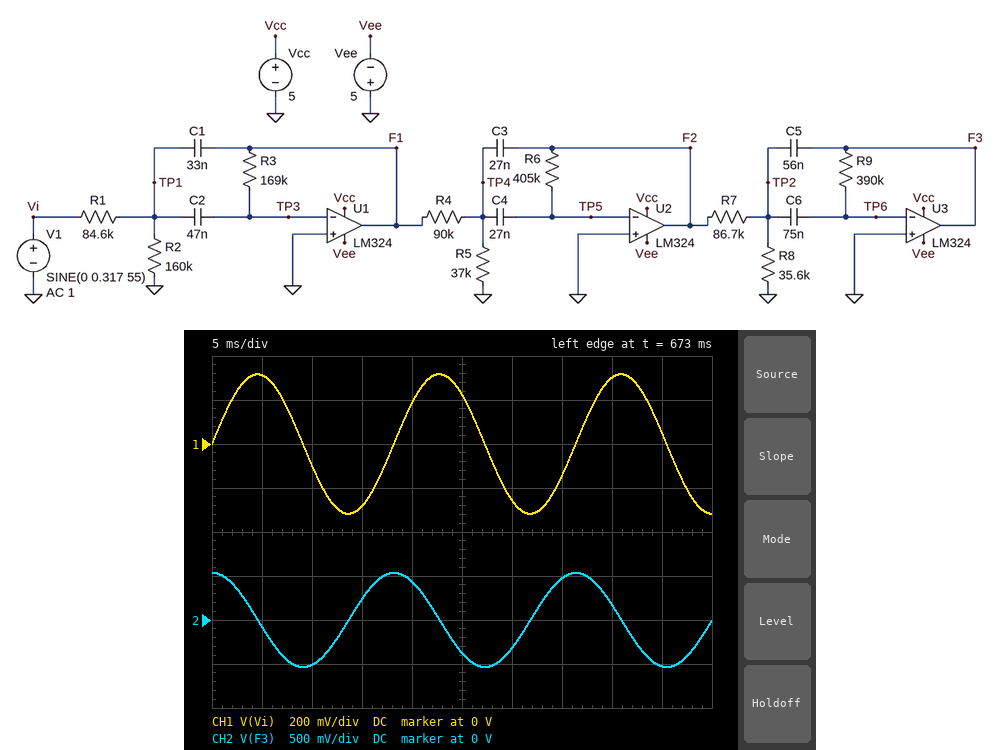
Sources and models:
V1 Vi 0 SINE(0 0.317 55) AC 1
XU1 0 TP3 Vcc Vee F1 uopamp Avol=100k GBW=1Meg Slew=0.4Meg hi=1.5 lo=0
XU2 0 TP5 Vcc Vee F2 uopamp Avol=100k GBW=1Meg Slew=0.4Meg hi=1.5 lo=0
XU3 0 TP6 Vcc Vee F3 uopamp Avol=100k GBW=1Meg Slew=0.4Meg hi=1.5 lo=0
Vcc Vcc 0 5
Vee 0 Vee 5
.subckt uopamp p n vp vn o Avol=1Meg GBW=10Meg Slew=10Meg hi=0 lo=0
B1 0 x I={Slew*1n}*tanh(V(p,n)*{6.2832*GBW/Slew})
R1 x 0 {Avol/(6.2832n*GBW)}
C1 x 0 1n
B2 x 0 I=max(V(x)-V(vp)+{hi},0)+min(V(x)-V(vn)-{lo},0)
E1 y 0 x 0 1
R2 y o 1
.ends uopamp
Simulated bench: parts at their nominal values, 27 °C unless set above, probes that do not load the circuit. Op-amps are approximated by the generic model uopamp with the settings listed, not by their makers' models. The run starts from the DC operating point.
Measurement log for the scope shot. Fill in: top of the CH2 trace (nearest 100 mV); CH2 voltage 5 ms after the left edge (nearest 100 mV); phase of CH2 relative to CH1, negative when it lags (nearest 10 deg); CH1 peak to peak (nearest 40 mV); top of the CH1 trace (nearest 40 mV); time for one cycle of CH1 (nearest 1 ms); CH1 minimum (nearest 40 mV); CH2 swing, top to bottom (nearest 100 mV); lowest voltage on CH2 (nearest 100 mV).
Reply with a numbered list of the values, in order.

1. 500 mV
2. -100 mV
3. 90 deg
4. 640 mV
5. 320 mV
6. 18 ms
7. -320 mV
8. 1.1 V
9. -500 mV
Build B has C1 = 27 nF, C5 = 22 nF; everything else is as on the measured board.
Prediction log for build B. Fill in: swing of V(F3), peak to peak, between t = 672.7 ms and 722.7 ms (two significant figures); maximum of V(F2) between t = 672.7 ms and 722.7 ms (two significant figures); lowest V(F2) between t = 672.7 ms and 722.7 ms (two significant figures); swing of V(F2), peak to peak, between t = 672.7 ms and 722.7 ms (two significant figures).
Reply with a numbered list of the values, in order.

1. 4.0 V
2. 860 mV
3. -860 mV
4. 1.7 V
